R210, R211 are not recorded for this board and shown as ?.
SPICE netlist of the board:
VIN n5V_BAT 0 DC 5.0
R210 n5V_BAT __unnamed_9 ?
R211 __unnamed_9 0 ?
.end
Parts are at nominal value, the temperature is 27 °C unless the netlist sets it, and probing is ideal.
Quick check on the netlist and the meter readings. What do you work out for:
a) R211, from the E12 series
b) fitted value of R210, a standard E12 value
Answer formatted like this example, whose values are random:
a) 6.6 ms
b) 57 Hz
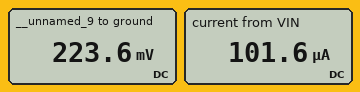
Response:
a) 2.2 kΩ
b) 47 kΩ
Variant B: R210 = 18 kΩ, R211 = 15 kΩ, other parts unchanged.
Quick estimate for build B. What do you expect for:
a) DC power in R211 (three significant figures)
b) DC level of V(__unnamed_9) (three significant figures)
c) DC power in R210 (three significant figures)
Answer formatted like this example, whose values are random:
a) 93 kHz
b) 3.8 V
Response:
a) 344 µW
b) 2.27 V
c) 413 µW
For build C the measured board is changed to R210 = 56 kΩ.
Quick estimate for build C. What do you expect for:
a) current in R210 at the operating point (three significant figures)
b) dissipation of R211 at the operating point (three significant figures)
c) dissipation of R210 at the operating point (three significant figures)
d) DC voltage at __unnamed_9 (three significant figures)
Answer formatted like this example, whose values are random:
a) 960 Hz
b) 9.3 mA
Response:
a) 85.9 µA
b) 16.2 µW
c) 413 µW
d) 189 mV
